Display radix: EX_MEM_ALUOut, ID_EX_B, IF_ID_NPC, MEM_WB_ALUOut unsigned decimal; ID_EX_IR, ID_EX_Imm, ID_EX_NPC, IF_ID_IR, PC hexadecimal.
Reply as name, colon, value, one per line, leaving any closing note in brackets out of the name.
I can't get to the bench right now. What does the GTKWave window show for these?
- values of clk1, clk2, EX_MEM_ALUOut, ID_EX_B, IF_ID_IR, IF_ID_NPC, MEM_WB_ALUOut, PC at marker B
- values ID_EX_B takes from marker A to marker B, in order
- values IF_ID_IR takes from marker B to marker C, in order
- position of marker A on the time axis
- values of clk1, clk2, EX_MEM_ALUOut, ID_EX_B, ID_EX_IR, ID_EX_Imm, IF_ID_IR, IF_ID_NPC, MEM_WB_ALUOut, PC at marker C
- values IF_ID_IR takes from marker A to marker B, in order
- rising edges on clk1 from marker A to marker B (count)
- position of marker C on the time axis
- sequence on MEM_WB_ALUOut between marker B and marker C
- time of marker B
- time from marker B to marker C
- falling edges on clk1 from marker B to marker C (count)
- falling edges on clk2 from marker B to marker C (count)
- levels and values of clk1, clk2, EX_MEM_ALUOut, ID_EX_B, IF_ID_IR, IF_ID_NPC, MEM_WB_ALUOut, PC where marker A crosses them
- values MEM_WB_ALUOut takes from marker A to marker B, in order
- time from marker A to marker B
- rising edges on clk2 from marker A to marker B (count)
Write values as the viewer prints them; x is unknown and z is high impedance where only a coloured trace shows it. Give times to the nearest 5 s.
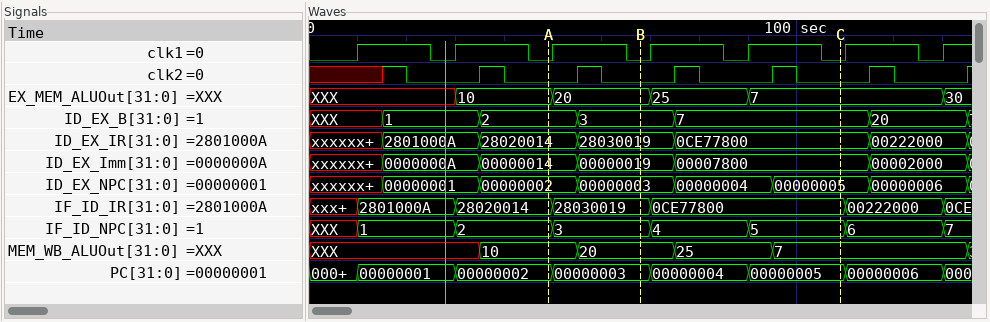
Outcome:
values of clk1, clk2, EX_MEM_ALUOut, ID_EX_B, IF_ID_IR, IF_ID_NPC, MEM_WB_ALUOut, PC at marker B: clk1=0, clk2=0, EX_MEM_ALUOut=20, ID_EX_B=3, IF_ID_IR=28030019, IF_ID_NPC=3, MEM_WB_ALUOut=20, PC=00000003
values ID_EX_B takes from marker A to marker B, in order: 2, 3
values IF_ID_IR takes from marker B to marker C, in order: 28030019, 0CE77800
position of marker A on the time axis: 50 s
values of clk1, clk2, EX_MEM_ALUOut, ID_EX_B, ID_EX_IR, ID_EX_Imm, IF_ID_IR, IF_ID_NPC, MEM_WB_ALUOut, PC at marker C: clk1=0, clk2=0, EX_MEM_ALUOut=7, ID_EX_B=7, ID_EX_IR=0CE77800, ID_EX_Imm=00007800, IF_ID_IR=0CE77800, IF_ID_NPC=5, MEM_WB_ALUOut=7, PC=00000005
values IF_ID_IR takes from marker A to marker B, in order: 28020014, 28030019
rising edges on clk1 from marker A to marker B: 1
position of marker C on the time axis: 110 s
sequence on MEM_WB_ALUOut between marker B and marker C: 20, 25, 7
time of marker B: 70 s
time from marker B to marker C: 40 s
falling edges on clk1 from marker B to marker C: 2
falling edges on clk2 from marker B to marker C: 2
levels and values of clk1, clk2, EX_MEM_ALUOut, ID_EX_B, IF_ID_IR, IF_ID_NPC, MEM_WB_ALUOut, PC where marker A crosses them: clk1=0, clk2=0, EX_MEM_ALUOut=10, ID_EX_B=2, IF_ID_IR=28020014, IF_ID_NPC=2, MEM_WB_ALUOut=10, PC=00000002
values MEM_WB_ALUOut takes from marker A to marker B, in order: 10, 20
time from marker A to marker B: 20 s
rising edges on clk2 from marker A to marker B: 1
